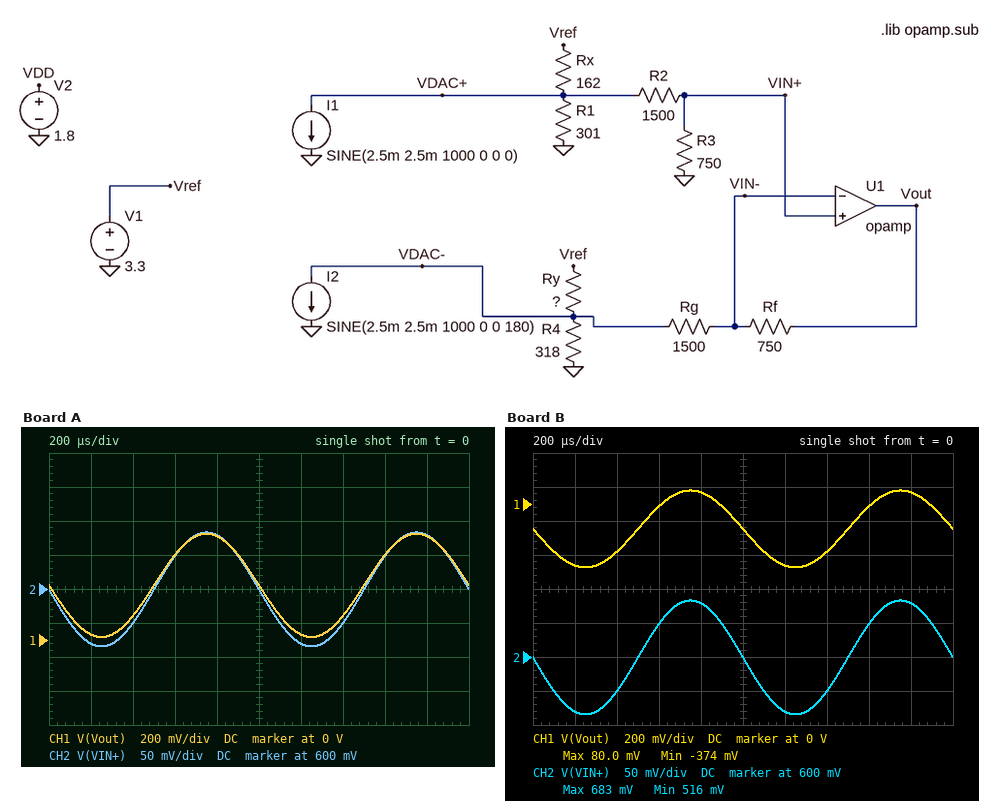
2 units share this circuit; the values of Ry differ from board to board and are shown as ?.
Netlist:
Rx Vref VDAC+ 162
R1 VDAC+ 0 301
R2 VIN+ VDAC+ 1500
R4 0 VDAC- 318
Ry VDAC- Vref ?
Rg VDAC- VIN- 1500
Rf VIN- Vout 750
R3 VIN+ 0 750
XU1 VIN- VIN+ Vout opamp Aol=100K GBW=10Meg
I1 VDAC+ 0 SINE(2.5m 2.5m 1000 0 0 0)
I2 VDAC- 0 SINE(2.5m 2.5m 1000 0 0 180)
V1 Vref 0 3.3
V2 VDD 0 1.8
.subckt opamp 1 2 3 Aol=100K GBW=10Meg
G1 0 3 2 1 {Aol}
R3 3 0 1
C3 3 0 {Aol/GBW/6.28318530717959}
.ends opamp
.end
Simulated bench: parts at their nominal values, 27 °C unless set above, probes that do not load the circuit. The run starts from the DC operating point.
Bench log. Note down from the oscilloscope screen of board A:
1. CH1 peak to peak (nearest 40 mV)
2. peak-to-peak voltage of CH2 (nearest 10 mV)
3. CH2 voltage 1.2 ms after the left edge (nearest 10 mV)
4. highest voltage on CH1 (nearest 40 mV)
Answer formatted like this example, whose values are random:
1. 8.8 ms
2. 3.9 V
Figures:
1. 600 mV
2. 170 mV
3. 520 mV
4. 640 mV
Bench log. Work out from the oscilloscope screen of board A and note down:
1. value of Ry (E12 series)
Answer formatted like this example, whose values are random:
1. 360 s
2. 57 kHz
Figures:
1. 330 Ω
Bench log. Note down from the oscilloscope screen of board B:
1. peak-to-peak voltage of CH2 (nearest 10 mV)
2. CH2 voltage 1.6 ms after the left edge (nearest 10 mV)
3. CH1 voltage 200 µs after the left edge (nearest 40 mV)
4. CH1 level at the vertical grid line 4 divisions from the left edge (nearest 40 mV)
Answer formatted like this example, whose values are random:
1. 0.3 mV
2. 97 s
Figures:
1. 170 mV
2. 650 mV
3. -360 mV
4. 80 mV
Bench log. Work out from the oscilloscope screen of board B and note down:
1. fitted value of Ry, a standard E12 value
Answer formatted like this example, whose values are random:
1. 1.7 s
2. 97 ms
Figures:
1. 120 Ω
